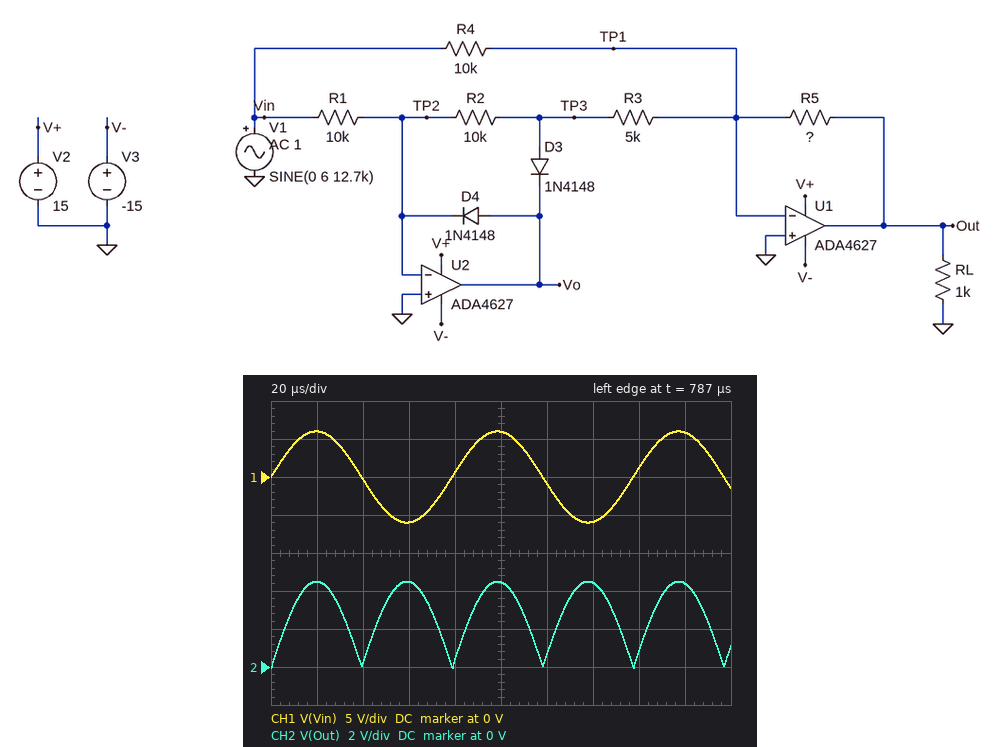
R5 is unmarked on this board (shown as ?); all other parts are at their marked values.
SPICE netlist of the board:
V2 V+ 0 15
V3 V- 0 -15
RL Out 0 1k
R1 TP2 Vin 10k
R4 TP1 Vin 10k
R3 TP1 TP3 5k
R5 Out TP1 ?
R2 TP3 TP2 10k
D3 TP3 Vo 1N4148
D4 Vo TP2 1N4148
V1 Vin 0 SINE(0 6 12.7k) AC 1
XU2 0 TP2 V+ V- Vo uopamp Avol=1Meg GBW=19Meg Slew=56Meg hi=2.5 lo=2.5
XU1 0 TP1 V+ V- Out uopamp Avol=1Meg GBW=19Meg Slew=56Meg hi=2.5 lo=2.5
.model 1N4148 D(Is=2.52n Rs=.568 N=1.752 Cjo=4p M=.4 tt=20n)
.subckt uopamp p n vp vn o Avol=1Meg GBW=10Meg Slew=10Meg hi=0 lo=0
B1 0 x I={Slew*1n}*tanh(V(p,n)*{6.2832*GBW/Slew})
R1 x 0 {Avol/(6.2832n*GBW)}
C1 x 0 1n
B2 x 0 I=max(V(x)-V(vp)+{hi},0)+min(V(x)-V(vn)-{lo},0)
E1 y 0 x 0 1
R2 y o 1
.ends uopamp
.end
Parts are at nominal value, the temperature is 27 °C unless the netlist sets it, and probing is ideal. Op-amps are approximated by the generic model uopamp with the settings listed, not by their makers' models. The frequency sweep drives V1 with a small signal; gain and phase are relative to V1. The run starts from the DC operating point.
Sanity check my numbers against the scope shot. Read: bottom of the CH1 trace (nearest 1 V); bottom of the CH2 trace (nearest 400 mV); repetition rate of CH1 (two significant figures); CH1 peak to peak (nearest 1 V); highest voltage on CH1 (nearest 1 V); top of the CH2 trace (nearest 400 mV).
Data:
-6 V
0 V
13 kHz
12 V
6 V
4.4 V
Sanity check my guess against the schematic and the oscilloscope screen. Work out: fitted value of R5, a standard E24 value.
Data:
7.5 kΩ
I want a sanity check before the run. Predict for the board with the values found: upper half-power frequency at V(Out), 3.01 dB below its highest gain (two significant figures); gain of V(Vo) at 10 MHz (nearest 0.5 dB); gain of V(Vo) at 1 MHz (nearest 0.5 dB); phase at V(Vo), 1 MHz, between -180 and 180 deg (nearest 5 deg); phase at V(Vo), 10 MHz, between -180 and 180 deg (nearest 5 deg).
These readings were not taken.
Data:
12 MHz
-11.5 dB
7.5 dB
90 deg
75 deg
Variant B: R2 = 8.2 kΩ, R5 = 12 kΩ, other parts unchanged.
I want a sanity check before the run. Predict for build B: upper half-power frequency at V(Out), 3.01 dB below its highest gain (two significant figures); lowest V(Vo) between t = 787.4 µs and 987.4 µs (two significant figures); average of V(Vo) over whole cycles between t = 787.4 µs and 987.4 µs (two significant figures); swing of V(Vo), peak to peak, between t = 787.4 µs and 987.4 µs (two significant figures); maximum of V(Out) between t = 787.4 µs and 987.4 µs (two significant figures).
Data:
7.3 MHz
-5.5 V
-1.6 V
6.1 V
7.2 V
